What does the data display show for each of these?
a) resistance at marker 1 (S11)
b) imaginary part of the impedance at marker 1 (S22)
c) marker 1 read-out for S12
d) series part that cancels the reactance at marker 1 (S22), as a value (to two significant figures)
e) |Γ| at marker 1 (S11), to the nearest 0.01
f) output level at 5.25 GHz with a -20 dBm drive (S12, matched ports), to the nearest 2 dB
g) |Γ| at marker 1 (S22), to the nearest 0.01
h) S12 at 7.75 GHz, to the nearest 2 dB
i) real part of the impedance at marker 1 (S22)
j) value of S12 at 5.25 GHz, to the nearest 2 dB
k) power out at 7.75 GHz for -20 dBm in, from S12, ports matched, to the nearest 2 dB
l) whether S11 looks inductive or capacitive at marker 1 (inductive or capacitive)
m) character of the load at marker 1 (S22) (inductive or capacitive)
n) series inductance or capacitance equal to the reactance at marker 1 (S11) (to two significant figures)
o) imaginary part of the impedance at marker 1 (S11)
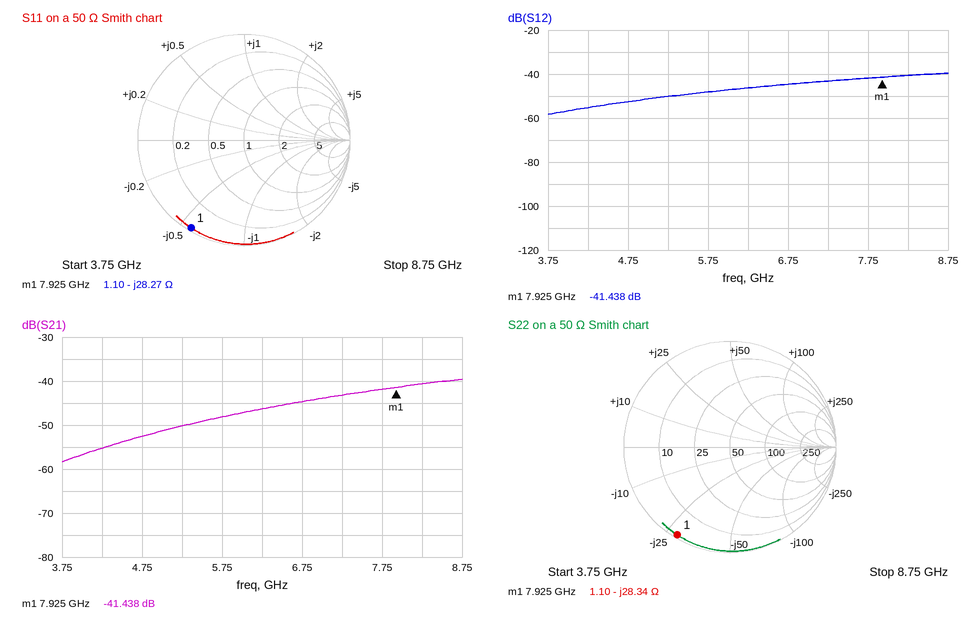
1.10 Ω
-28.34 Ω
-41.438 dB
570 pH
0.97
-70 dBm
0.97
-42 dB
1.10 Ω
-50 dB
-62 dBm
capacitive
capacitive
710 fF
-28.27 Ω
